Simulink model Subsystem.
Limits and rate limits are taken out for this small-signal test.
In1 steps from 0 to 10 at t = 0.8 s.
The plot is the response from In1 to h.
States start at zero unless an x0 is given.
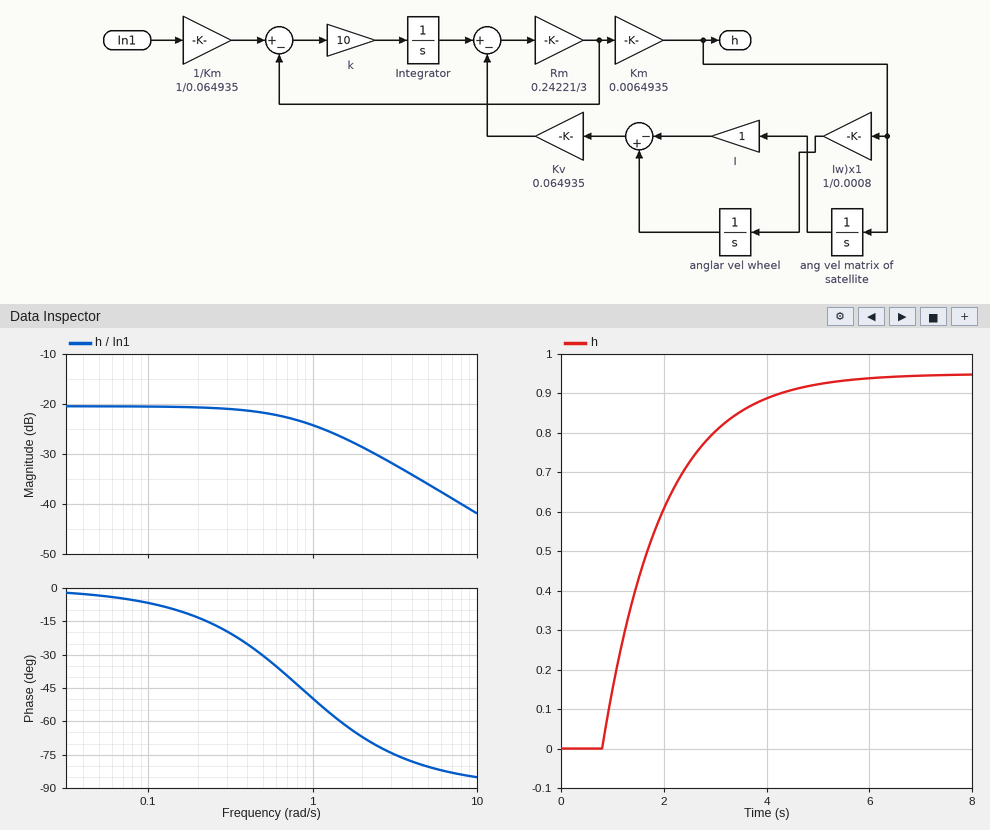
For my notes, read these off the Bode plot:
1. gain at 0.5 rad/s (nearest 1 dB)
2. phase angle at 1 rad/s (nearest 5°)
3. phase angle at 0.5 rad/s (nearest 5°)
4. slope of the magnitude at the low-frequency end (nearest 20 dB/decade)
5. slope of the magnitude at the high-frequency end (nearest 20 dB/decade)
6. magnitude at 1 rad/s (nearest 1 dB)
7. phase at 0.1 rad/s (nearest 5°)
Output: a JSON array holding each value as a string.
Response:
["-22 dB", "-50°", "-30°", "0 dB/decade", "-20 dB/decade", "-24 dB", "-5°"]
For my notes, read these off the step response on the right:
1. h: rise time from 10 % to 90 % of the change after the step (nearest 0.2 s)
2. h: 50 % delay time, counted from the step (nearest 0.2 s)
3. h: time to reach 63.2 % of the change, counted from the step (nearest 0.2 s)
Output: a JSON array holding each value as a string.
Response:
["2.6 s", "0.8 s", "1.2 s"]
